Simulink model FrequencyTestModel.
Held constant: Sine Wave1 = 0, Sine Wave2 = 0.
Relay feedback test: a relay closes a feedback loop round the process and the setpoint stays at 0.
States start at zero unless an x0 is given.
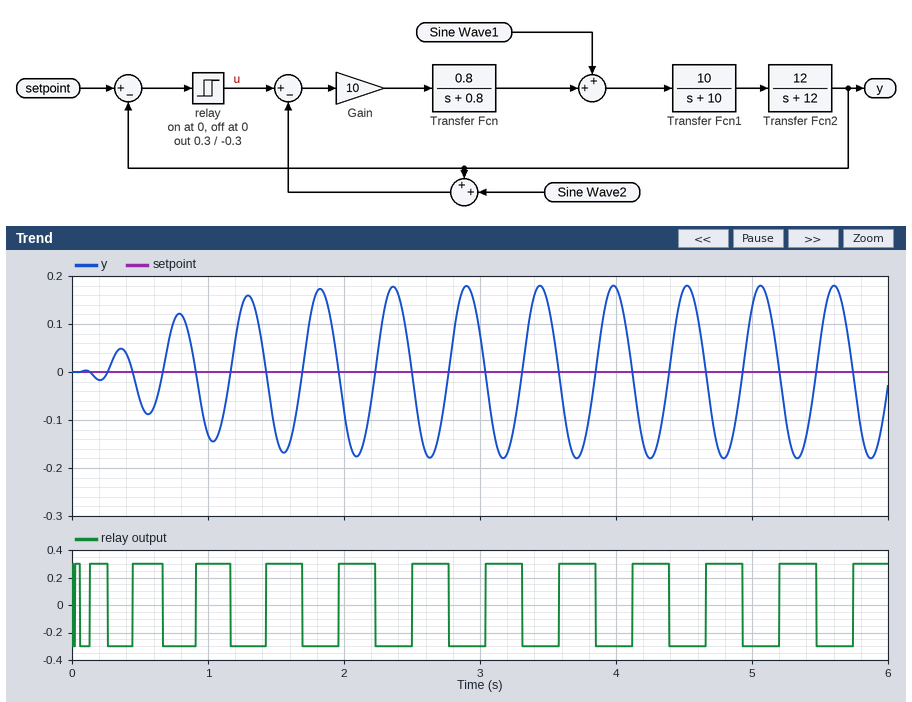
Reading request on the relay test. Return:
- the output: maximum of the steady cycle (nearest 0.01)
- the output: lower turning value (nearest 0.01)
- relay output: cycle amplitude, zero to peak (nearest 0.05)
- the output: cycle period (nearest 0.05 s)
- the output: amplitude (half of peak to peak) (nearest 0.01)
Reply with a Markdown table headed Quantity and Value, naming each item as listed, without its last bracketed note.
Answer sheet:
| Quantity | Value |
|---|---|
| the output: maximum of the steady cycle | 0.18 |
| the output: lower turning value | -0.18 |
| relay output: cycle amplitude, zero to peak | 0.30 |
| the output: cycle period | 0.55 s |
| the output: amplitude (half of peak to peak) | 0.18 |
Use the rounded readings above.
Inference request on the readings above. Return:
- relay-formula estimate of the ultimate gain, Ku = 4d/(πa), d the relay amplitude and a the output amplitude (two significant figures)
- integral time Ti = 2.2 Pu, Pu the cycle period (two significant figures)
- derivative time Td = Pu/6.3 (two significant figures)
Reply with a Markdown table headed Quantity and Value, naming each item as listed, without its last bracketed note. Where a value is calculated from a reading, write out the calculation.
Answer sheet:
| Quantity | Value |
|---|---|
| relay-formula estimate of the ultimate gain, Ku = 4d/(πa), d the relay amplitude and a the output amplitude | 4 × 0.3 / (π × 0.18) = 2.1 |
| integral time Ti = 2.2 Pu, Pu the cycle period | 2.2 × 0.55 = 1.2 s |
| derivative time Td = Pu/6.3 | 0.55 / 6.3 = 0.087 s |
